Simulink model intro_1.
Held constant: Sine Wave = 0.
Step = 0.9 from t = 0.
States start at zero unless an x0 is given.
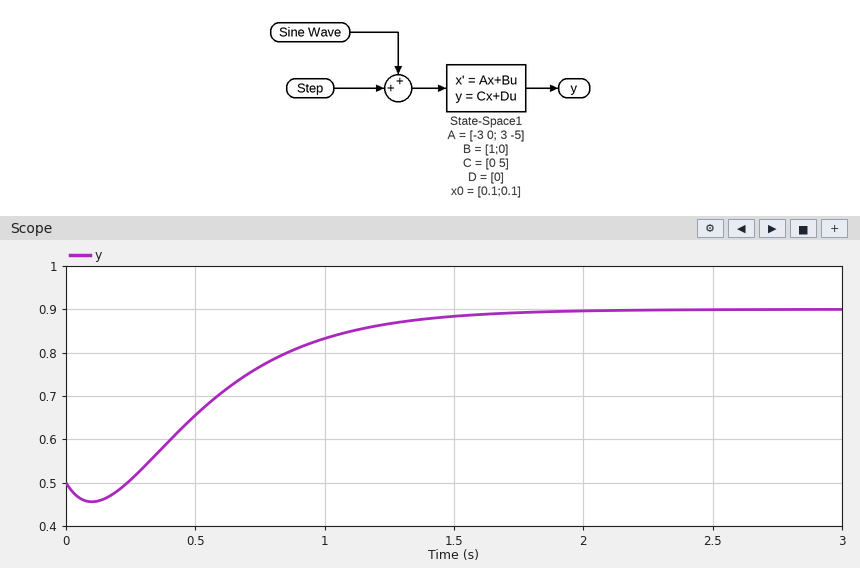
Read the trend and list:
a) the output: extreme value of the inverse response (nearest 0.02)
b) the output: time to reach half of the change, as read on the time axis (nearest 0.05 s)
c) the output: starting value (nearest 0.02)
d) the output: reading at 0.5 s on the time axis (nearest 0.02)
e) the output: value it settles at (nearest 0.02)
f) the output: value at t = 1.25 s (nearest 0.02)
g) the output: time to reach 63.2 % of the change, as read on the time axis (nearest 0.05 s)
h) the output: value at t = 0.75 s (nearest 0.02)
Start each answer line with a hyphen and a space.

- 0.46
- 0.60 s
- 0.50
- 0.66
- 0.90
- 0.86
- 0.70 s
- 0.76
